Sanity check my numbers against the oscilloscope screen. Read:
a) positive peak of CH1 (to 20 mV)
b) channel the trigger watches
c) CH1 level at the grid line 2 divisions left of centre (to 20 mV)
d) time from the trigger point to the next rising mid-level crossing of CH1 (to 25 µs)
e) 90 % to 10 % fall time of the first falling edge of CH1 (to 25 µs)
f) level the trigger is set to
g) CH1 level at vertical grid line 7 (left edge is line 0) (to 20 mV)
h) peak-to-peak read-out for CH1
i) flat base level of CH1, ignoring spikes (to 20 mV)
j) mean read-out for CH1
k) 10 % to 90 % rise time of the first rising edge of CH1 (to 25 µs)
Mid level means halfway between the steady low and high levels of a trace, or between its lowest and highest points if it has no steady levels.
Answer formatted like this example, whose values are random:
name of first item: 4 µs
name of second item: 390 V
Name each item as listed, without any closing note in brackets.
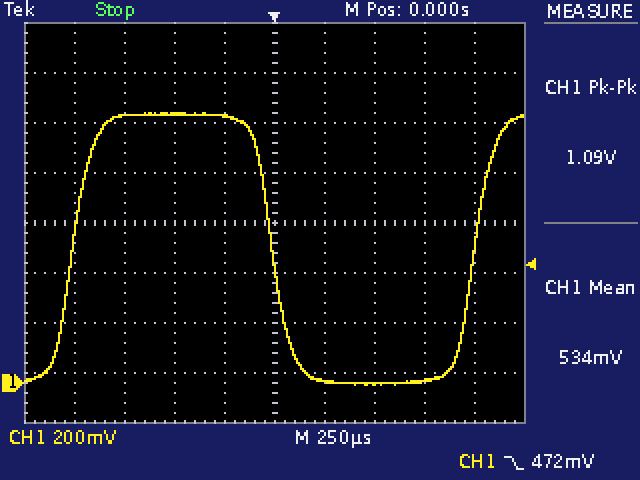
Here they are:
positive peak of CH1: 1.08 V
channel the trigger watches: CH1
CH1 level at the grid line 2 divisions left of centre: 1.08 V
time from the trigger point to the next rising mid-level crossing of CH1: 1.000 ms
90 % to 10 % fall time of the first falling edge of CH1: 200 µs
level the trigger is set to: 472 mV
CH1 level at vertical grid line 7 (left edge is line 0): 0 mV
peak-to-peak read-out for CH1: 1.09 V
flat base level of CH1, ignoring spikes: 0 mV
mean read-out for CH1: 534 mV
10 % to 90 % rise time of the first rising edge of CH1: 200 µs
